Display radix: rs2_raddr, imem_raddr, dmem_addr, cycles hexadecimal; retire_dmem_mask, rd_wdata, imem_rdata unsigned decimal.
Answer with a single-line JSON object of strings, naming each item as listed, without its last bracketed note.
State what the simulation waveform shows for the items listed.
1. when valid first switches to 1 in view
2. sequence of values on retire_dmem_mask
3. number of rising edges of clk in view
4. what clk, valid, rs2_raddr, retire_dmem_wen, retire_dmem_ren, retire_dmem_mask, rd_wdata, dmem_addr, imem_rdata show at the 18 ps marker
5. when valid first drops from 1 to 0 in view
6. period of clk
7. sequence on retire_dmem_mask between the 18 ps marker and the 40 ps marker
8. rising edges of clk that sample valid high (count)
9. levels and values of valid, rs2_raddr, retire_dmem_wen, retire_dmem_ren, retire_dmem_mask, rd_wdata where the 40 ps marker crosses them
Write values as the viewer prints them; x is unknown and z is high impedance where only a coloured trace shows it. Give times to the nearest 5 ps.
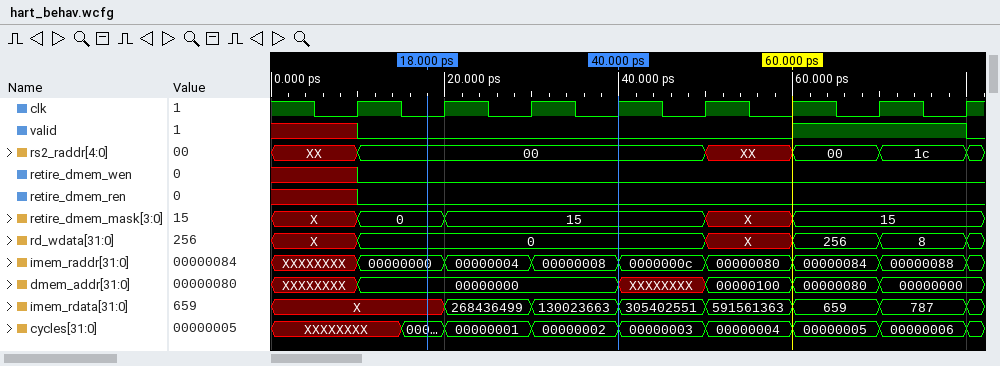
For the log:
{"when valid first switches to 1 in view": "60 ps", "sequence of values on retire_dmem_mask": "X, 0, 15, X, 15", "number of rising edges of clk in view": "8", "what clk, valid, rs2_raddr, retire_dmem_wen, retire_dmem_ren, retire_dmem_mask, rd_wdata, dmem_addr, imem_rdata show at the 18 ps marker": "clk=0, valid=0, rs2_raddr=00, retire_dmem_wen=0, retire_dmem_ren=0, retire_dmem_mask=0, rd_wdata=0, dmem_addr=00000000, imem_rdata=X", "when valid first drops from 1 to 0 in view": "80 ps", "period of clk": "10 ps", "sequence on retire_dmem_mask between the 18 ps marker and the 40 ps marker": "0, 15", "rising edges of clk that sample valid high": "2", "levels and values of valid, rs2_raddr, retire_dmem_wen, retire_dmem_ren, retire_dmem_mask, rd_wdata where the 40 ps marker crosses them": "valid=0, rs2_raddr=00, retire_dmem_wen=0, retire_dmem_ren=0, retire_dmem_mask=15, rd_wdata=0"}
